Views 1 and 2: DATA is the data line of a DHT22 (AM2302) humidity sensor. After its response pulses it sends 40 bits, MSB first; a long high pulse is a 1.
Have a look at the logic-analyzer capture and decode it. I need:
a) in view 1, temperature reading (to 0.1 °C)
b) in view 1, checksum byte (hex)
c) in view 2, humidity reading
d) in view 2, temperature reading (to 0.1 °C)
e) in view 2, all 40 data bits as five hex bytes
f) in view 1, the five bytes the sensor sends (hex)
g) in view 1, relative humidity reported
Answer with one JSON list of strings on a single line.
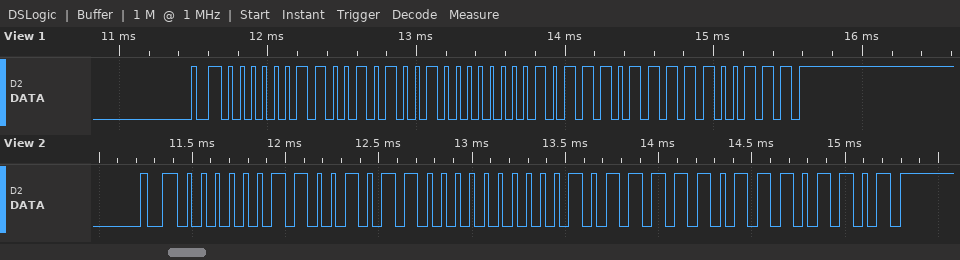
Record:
["18.7 °C", "0xE7", "81.2 %", "19.0 °C", "03 2C 00 BE ED", "03 29 00 BB E7", "80.9 %"]
